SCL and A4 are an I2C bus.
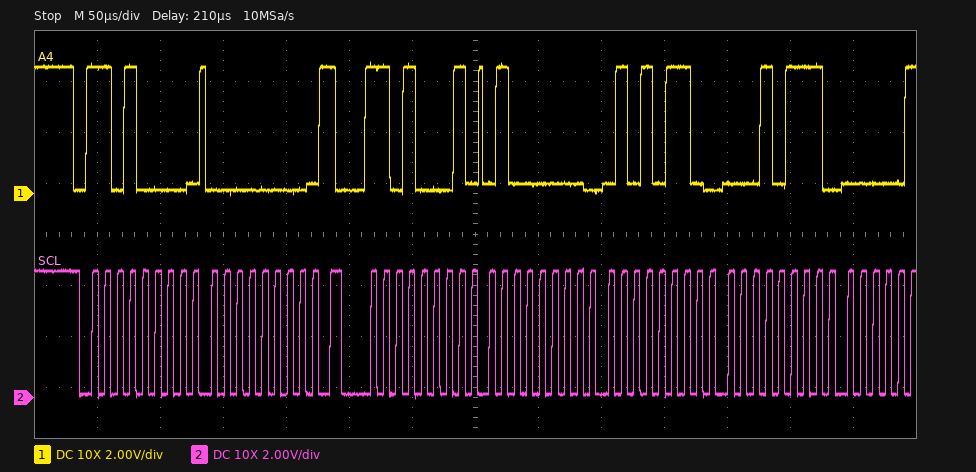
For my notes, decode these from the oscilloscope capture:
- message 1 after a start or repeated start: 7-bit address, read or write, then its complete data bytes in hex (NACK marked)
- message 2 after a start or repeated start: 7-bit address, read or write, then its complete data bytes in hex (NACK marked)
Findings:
0x68 write: 00
0x68 read: 40 56 17
